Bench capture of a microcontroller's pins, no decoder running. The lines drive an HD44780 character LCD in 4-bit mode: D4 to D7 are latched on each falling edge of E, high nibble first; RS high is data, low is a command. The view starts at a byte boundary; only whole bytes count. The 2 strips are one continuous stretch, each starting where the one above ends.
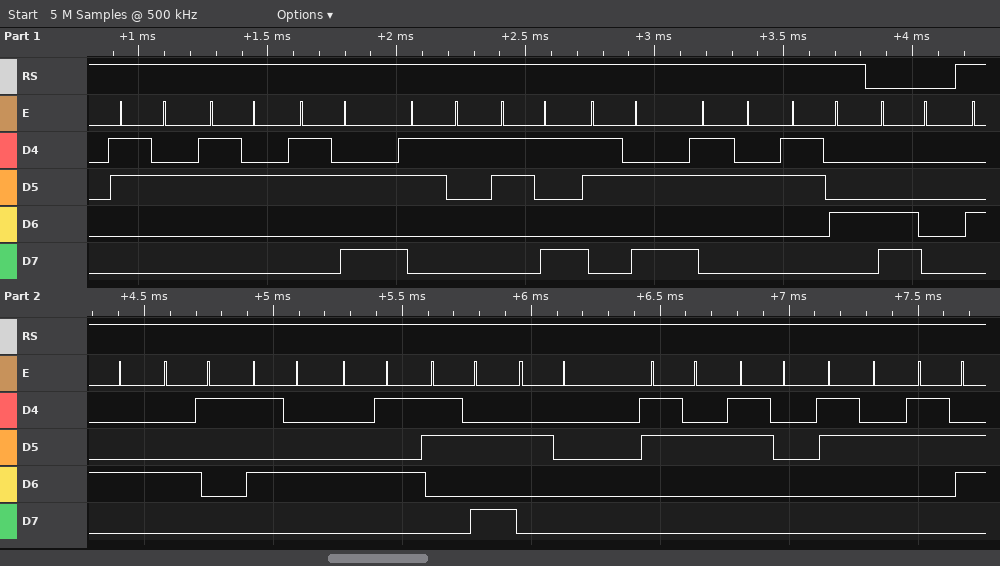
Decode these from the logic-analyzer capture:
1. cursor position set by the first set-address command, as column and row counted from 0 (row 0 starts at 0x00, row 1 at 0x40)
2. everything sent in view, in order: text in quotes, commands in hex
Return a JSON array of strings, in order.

["column 0, row 1", "\"22:19:24\" 0xC0 \"DATE: 2026\""]
